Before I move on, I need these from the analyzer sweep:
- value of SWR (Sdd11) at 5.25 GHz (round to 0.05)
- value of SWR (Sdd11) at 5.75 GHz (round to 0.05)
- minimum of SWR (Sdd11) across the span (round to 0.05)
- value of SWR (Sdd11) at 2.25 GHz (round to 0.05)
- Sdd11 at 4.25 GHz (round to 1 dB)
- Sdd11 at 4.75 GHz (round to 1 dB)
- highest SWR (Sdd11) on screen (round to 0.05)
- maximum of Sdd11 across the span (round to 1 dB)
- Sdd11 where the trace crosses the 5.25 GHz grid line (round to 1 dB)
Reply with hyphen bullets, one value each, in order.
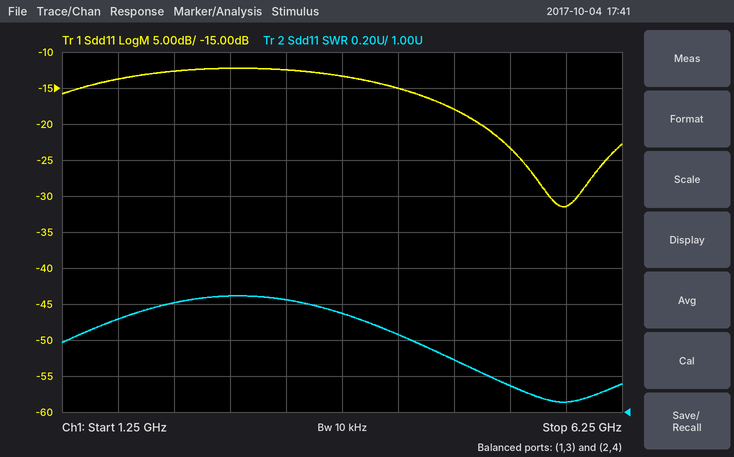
- 1.15
- 1.05
- 1.05
- 1.60
- -15 dB
- -18 dB
- 1.65
- -12 dB
- -23 dB
